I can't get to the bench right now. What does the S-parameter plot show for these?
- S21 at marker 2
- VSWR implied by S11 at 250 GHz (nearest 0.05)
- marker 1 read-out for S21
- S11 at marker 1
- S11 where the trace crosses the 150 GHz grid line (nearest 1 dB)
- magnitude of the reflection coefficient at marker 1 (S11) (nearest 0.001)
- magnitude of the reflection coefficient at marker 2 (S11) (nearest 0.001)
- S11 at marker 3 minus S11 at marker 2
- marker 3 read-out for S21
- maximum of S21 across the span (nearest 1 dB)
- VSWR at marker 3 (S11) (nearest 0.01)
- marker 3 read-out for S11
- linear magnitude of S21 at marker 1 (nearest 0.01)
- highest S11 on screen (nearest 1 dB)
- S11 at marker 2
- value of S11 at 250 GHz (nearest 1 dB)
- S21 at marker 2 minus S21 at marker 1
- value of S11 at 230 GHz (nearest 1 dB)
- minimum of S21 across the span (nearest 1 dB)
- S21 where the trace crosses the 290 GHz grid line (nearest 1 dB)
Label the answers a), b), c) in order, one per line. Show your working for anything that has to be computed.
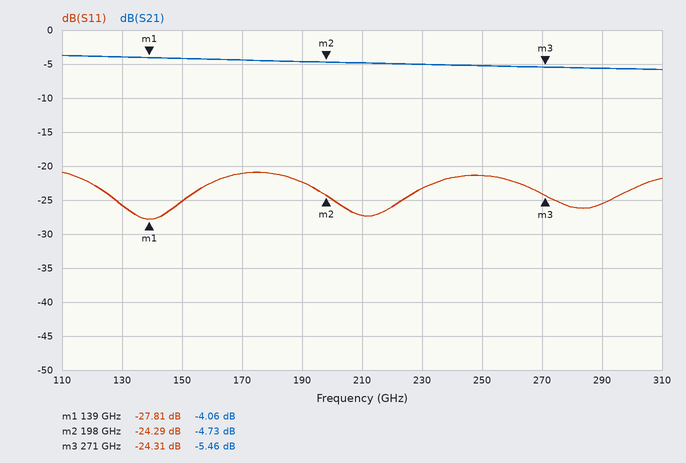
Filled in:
a) -4.73 dB
b) |Γ| = 10^(-21/20) = 0.0891; VSWR = (1 + 0.0891)/(1 − 0.0891) ≈ 1.20
c) -4.06 dB
d) -27.81 dB
e) -25 dB
f) 10^(-27.81/20) ≈ 0.041
g) 10^(-24.29/20) ≈ 0.061
h) -24.31 − (-24.29) = -0.02 dB
i) -5.46 dB
j) -4 dB
k) (1 + 0.0609)/(1 − 0.0609) ≈ 1.13
l) -24.31 dB
m) 10^(-4.06/20) ≈ 0.63
n) -21 dB
o) -24.29 dB
p) -21 dB
q) -4.73 − (-4.06) = -0.67 dB
r) -23 dB
s) -6 dB
t) -6 dB
